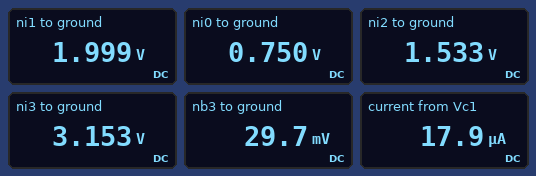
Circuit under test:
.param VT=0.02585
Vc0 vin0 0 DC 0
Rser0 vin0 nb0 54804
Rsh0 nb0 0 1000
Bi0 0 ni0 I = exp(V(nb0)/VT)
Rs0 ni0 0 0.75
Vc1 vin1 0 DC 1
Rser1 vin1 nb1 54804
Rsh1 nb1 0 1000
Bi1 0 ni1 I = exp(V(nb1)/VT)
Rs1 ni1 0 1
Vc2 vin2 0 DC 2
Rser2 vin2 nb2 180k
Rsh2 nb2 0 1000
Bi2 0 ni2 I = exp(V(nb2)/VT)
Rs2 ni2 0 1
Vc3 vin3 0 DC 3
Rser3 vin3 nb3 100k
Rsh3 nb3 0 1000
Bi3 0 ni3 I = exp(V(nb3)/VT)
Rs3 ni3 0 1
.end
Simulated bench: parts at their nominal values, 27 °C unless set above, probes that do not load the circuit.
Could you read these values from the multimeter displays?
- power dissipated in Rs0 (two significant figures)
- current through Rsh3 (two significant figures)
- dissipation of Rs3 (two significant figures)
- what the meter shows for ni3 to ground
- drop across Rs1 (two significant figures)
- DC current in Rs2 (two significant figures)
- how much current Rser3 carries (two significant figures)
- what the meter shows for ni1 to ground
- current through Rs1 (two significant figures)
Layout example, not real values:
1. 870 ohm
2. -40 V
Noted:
1. 750 mW
2. 30 µA
3. 9.9 W
4. 3.153 V
5. 2.0 V
6. 1.5 A
7. 30 µA
8. 1.999 V
9. 2.0 A
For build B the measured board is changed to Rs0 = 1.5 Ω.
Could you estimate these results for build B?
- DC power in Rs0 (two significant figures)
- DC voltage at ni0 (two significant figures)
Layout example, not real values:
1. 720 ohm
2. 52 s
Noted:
1. 1.5 W
2. 1.5 V
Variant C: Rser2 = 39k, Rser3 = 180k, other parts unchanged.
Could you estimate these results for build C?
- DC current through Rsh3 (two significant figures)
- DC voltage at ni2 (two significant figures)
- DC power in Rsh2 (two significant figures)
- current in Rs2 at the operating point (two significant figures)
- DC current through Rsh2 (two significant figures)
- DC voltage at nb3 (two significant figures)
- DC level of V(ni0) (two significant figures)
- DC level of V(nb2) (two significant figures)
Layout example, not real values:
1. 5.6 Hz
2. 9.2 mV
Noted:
1. 17 µA
2. 6.9 V
3. 2.5 µW
4. 6.9 A
5. 50 µA
6. 17 mV
7. 750 mV
8. 50 mV
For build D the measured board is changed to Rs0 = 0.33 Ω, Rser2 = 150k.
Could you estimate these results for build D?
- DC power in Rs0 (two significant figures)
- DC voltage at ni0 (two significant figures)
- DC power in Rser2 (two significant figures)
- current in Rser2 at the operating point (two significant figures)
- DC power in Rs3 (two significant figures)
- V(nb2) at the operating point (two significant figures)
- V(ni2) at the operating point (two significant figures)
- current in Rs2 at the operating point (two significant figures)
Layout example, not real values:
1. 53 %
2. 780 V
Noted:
1. 330 mW
2. 330 mV
3. 26 µW
4. 13 µA
5. 9.9 W
6. 13 mV
7. 1.7 V
8. 1.7 A
